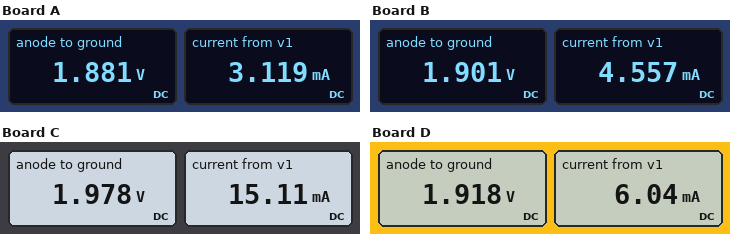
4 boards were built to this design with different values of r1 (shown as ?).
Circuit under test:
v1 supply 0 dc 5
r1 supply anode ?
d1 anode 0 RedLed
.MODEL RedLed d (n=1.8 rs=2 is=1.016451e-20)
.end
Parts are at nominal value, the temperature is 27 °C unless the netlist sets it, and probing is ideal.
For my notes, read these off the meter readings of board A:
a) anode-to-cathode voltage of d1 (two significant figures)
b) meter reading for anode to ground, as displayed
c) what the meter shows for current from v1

1.9 V
1.881 V
3.119 mA
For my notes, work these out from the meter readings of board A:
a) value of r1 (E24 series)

1 kΩ
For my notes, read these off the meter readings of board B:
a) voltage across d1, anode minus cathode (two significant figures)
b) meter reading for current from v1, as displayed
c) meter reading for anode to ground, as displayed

1.9 V
4.557 mA
1.901 V
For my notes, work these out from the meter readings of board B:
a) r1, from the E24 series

680 Ω
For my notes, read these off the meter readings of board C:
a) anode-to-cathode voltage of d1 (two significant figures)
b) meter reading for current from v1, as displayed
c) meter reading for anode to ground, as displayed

2.0 V
15.11 mA
1.978 V
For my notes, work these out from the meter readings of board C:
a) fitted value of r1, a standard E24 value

200 Ω
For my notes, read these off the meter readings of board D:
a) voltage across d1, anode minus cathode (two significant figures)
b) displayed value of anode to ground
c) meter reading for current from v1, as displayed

1.9 V
1.918 V
6.04 mA
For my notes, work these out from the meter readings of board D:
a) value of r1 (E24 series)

510 Ω
